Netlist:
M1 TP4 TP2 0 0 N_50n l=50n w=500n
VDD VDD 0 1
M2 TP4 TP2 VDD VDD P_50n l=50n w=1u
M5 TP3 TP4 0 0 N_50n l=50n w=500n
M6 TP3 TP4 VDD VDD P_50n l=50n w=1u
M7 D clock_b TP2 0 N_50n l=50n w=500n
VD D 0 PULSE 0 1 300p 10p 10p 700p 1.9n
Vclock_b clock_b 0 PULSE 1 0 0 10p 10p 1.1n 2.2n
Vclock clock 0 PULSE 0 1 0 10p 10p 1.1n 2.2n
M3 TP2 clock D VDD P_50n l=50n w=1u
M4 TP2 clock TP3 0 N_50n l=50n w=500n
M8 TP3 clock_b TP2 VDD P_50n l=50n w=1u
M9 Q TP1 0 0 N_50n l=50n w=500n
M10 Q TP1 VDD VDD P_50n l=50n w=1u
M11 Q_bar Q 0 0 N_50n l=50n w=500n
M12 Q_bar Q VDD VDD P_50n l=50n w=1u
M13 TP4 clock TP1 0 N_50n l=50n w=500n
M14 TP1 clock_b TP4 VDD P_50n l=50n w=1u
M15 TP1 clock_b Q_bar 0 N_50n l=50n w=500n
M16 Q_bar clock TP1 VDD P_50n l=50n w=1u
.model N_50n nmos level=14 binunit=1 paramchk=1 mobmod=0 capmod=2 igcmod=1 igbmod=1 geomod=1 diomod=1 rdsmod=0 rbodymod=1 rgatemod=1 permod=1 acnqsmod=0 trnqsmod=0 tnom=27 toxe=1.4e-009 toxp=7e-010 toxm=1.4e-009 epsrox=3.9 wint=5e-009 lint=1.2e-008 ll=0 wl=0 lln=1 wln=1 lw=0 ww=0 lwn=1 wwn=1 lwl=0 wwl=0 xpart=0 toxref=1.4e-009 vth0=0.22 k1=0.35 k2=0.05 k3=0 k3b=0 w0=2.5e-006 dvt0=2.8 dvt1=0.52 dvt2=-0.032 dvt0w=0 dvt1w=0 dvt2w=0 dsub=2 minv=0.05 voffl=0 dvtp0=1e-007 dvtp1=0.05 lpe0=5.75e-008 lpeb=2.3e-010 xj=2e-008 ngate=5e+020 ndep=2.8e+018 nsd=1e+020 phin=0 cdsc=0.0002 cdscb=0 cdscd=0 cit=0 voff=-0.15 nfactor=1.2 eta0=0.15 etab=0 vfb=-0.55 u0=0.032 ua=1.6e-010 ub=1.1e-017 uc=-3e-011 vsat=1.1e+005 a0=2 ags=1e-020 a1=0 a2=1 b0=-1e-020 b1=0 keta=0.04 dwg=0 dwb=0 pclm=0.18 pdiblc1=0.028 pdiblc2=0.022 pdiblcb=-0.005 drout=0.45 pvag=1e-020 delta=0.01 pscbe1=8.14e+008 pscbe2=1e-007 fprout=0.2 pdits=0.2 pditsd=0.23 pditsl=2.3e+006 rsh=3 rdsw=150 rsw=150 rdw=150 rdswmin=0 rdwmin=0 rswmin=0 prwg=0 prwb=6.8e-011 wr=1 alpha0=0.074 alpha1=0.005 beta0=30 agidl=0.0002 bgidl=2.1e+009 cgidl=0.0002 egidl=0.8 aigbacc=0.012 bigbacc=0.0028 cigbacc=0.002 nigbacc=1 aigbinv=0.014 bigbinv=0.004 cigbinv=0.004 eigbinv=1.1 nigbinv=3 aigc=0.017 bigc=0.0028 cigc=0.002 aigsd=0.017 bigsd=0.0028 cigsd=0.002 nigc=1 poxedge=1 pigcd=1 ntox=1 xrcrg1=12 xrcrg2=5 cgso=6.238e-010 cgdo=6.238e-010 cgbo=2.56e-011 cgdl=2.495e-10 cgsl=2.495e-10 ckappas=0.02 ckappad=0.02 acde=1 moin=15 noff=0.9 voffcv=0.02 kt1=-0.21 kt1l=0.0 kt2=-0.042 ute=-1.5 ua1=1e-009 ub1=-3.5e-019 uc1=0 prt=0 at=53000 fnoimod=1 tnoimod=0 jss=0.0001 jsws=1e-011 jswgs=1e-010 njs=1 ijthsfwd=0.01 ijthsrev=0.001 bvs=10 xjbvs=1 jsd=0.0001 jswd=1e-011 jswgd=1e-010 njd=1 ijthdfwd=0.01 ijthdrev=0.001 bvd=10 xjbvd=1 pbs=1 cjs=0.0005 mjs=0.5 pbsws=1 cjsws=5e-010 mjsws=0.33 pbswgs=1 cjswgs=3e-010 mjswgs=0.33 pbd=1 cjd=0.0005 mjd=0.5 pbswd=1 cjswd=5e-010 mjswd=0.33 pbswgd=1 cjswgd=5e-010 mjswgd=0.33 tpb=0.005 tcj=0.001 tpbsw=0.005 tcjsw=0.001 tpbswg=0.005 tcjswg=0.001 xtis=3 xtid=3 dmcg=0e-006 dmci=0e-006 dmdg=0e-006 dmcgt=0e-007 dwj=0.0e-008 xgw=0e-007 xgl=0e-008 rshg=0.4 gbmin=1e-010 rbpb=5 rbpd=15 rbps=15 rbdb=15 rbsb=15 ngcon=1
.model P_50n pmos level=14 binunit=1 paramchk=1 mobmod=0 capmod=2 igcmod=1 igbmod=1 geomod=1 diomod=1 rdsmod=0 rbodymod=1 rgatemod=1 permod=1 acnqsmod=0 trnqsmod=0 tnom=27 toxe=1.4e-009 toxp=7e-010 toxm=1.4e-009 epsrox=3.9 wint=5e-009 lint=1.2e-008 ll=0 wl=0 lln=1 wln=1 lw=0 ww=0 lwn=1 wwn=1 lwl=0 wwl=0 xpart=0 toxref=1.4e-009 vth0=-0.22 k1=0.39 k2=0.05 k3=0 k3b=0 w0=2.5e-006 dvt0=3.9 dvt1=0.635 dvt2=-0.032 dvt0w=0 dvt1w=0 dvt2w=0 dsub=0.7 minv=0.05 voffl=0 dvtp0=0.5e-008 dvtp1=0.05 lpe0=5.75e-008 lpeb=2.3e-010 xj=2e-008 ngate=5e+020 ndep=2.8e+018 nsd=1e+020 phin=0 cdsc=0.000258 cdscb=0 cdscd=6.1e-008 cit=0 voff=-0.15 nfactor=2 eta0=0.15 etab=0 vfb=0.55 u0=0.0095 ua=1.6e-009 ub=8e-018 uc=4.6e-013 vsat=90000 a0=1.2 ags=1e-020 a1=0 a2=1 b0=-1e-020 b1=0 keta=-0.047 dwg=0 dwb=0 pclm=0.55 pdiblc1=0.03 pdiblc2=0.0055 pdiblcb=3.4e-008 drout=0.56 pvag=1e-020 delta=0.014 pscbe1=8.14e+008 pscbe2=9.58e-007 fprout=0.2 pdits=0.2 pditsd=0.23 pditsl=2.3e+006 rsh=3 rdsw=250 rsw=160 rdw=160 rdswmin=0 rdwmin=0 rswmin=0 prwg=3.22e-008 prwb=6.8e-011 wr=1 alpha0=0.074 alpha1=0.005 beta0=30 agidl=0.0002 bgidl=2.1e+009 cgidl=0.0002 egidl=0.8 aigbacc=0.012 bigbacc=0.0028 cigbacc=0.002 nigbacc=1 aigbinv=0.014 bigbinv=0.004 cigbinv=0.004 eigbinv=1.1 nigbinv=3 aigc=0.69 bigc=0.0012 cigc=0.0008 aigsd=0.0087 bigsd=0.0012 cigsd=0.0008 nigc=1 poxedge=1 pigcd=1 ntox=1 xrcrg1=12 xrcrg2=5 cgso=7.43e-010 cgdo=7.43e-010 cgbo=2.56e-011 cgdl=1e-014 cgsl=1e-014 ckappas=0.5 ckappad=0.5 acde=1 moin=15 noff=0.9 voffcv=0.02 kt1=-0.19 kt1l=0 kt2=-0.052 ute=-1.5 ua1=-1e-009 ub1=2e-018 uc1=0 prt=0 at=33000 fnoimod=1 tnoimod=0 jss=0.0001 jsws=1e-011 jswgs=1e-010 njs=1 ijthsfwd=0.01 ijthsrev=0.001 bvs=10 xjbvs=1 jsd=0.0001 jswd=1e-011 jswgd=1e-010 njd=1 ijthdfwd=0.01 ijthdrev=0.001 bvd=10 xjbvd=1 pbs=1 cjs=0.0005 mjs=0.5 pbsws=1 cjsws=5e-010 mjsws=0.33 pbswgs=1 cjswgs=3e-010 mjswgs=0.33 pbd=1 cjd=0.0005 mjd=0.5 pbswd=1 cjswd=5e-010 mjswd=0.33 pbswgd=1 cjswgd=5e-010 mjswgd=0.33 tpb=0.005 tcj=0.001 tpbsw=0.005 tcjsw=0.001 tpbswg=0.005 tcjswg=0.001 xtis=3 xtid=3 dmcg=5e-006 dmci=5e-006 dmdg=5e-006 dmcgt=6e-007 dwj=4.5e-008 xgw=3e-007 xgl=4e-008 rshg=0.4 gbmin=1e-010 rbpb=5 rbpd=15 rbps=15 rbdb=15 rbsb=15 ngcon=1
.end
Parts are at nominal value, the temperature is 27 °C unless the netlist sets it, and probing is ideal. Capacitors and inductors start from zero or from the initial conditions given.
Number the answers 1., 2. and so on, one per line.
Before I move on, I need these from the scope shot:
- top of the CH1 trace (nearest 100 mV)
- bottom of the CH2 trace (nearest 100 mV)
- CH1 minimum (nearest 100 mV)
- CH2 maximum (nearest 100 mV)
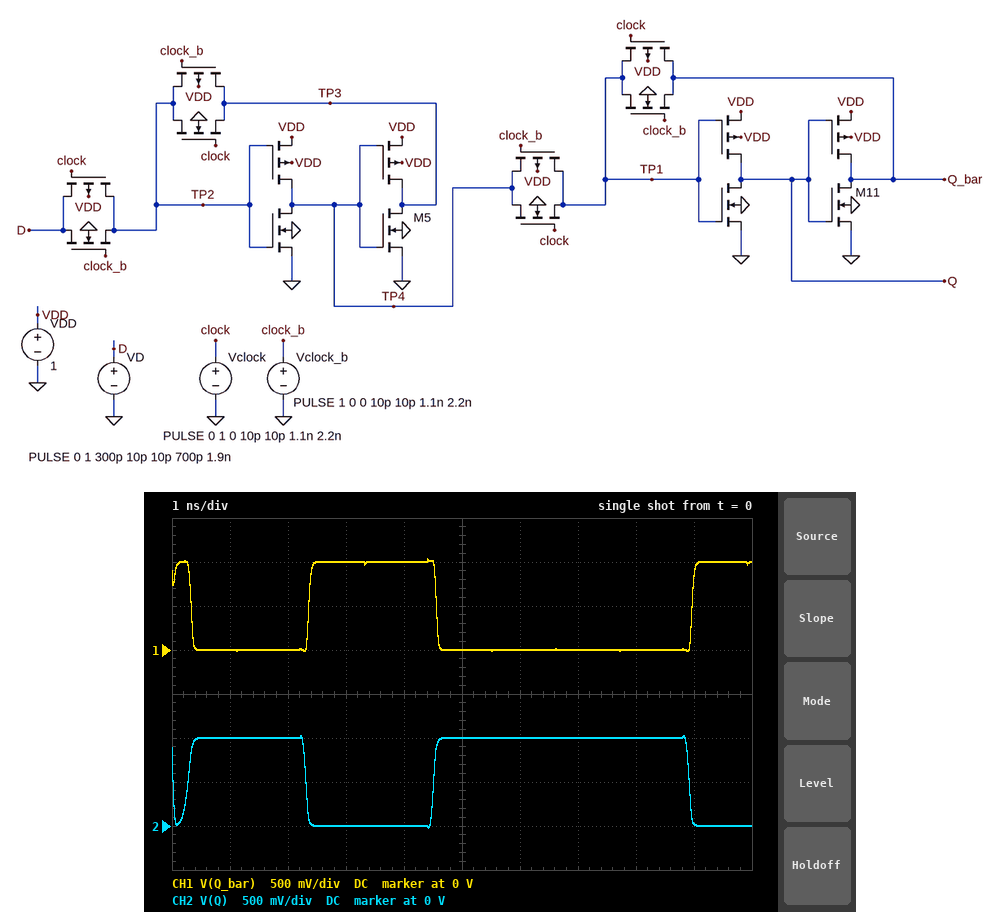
1. 1.0 V
2. 0 V
3. 0 V
4. 1.0 V
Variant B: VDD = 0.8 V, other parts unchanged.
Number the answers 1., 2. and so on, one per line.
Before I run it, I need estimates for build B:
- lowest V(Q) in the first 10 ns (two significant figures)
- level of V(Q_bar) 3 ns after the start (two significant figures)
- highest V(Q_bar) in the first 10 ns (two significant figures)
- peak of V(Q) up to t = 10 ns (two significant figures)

1. -18 mV
2. 800 mV
3. 830 mV
4. 820 mV
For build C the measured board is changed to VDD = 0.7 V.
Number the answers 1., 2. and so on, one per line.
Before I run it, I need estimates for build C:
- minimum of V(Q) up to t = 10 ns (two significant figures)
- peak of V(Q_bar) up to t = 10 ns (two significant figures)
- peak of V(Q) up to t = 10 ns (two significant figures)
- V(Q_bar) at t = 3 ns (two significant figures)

1. -19 mV
2. 730 mV
3. 720 mV
4. 700 mV
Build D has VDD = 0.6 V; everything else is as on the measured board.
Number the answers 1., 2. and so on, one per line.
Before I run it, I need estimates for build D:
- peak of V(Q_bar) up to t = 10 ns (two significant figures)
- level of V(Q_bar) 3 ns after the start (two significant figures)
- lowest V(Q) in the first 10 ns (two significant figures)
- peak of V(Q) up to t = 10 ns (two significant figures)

1. 630 mV
2. 600 mV
3. -22 mV
4. 610 mV
